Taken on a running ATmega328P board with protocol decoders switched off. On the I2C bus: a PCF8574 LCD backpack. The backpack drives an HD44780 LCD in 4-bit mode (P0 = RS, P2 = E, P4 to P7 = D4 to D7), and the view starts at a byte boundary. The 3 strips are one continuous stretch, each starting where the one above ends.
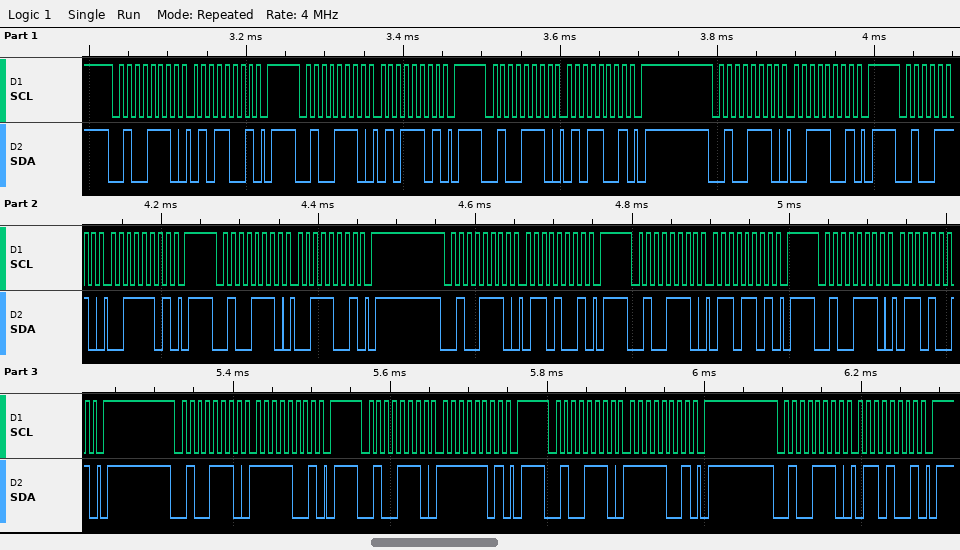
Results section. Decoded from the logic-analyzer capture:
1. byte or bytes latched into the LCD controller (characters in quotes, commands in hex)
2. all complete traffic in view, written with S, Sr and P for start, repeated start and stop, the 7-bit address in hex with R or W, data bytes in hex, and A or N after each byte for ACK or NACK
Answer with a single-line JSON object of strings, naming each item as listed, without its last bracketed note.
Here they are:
{"byte or bytes latched into the LCD controller": "'S' 'o'", "all complete traffic in view, written with S, Sr and P for start, repeated start and stop, the 7-bit address in hex with R or W, data bytes in hex, and A or N after each byte for ACK or NACK": "S 27W A 59 A P S 27W A 5D A P S 27W A 59 A P S 27W A 39 A P S 27W A 3D A P S 27W A 39 A P S 27W A 69 A P S 27W A 6D A P S 27W A 69 A P S 27W A F9 A P S 27W A FD A P S 27W A F9 A P S 27W A 69 A P"}
